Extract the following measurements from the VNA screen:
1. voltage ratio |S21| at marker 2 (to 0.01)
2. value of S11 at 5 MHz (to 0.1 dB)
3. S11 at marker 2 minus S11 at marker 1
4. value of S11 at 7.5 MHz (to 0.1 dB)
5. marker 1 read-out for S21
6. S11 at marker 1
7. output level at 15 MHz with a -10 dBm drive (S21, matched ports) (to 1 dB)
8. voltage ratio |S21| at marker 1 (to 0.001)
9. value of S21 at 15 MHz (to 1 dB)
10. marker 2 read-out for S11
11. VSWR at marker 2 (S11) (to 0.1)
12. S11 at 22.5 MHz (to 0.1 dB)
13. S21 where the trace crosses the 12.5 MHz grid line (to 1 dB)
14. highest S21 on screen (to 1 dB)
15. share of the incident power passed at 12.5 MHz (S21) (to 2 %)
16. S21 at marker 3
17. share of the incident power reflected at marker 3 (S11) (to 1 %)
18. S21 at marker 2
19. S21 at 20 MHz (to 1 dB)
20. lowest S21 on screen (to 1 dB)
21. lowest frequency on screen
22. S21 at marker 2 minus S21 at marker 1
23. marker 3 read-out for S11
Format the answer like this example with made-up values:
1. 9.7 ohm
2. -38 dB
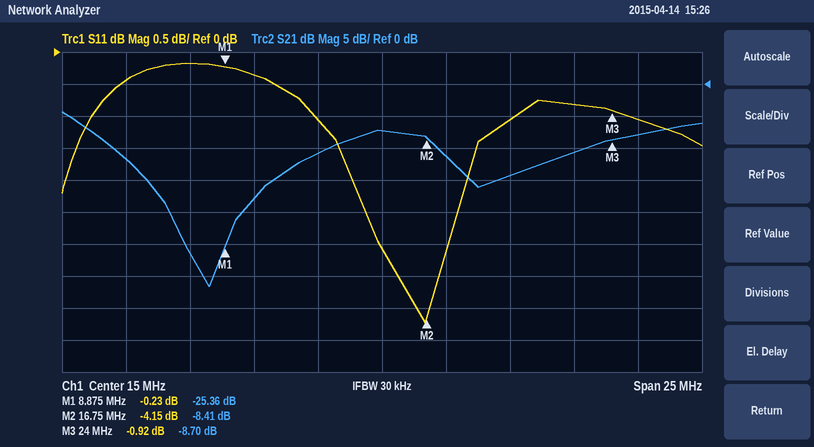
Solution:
1. 0.38
2. -0.4 dB
3. -3.92 dB
4. -0.2 dB
5. -25.36 dB
6. -0.23 dB
7. -17 dBm
8. 0.054
9. -7 dB
10. -4.15 dB
11. 4.3
12. -0.8 dB
13. -11 dB
14. -4 dB
15. 8 %
16. -8.70 dB
17. 81 %
18. -8.41 dB
19. -14 dB
20. -32 dB
21. 2.5 MHz
22. 16.95 dB
23. -0.92 dB
